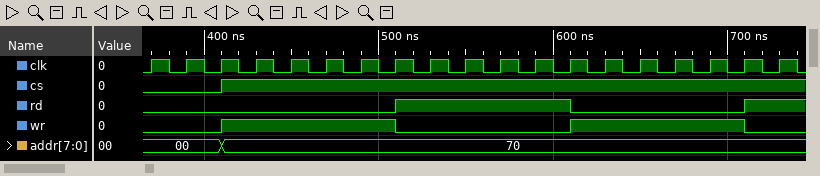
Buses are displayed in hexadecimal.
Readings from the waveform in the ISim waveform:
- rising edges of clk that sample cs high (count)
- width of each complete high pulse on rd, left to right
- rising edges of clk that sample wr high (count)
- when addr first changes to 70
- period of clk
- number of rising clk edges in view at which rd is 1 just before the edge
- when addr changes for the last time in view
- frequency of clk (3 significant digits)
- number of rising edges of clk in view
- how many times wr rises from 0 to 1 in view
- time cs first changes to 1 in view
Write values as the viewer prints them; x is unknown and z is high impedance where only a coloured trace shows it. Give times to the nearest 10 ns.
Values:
16
100 ns
10
410 ns
20 ns
6
410 ns
50.0 MHz
19
2
410 ns
